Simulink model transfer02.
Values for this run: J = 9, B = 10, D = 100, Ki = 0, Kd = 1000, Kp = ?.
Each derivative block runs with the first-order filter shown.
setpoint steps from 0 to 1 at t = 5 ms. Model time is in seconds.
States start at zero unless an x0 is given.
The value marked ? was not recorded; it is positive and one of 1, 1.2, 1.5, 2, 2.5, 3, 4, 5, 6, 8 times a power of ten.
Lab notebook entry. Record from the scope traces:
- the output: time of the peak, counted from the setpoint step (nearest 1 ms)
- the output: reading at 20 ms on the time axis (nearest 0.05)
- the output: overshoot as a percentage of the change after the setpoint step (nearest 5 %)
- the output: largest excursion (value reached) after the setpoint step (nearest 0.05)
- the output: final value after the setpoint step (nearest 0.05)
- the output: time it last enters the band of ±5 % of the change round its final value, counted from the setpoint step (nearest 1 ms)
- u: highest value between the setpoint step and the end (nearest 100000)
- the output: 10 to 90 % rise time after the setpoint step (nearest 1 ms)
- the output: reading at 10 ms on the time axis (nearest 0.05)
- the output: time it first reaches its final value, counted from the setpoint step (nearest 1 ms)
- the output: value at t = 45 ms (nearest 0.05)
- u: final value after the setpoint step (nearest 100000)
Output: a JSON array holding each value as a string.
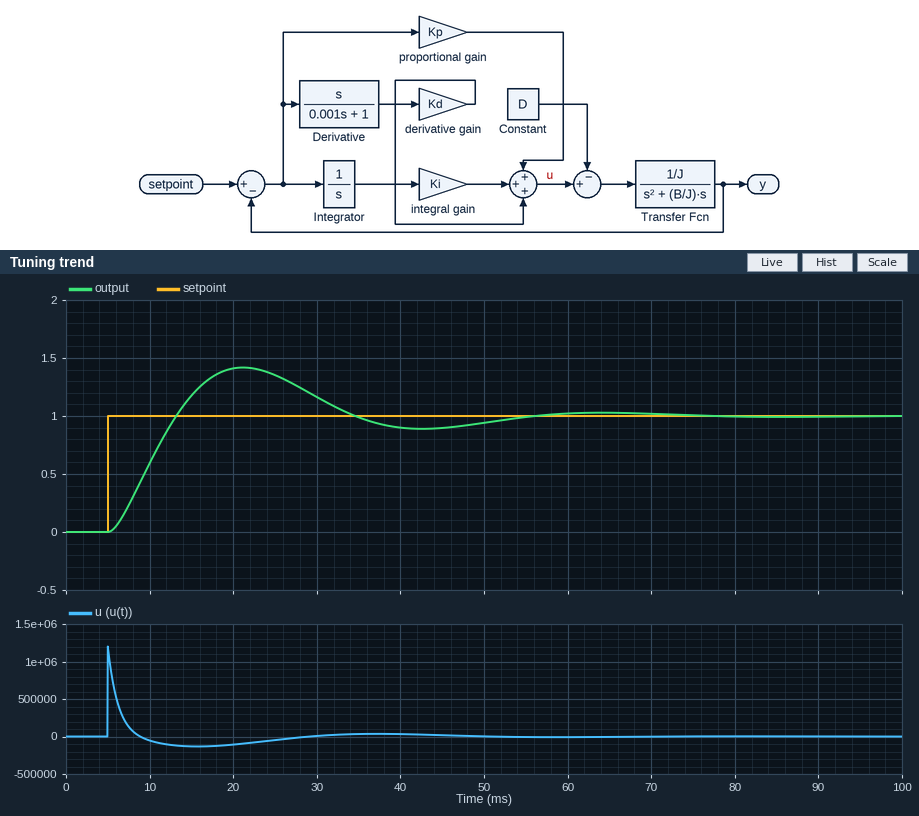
["16 ms", "1.40", "40 %", "1.40", "1.00", "46 ms", "1200000", "6 ms", "0.60", "8 ms", "0.90", "0"]
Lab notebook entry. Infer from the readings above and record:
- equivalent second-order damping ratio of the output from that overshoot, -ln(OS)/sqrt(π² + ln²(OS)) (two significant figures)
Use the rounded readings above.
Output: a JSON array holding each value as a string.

["0.28"]
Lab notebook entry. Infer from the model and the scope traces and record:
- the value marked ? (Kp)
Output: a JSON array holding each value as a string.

["200000"]
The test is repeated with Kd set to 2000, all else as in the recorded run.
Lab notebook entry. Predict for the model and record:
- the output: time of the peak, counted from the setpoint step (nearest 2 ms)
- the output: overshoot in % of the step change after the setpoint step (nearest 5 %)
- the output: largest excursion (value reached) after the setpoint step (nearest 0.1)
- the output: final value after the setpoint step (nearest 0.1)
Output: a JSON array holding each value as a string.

["12 ms", "25 %", "1.2", "1.0"]
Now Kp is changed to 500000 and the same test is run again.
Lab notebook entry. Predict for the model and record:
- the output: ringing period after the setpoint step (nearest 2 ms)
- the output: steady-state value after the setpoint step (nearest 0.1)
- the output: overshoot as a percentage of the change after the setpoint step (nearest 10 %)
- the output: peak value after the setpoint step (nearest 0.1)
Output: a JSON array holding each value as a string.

["26 ms", "1.0", "60 %", "1.6"]
